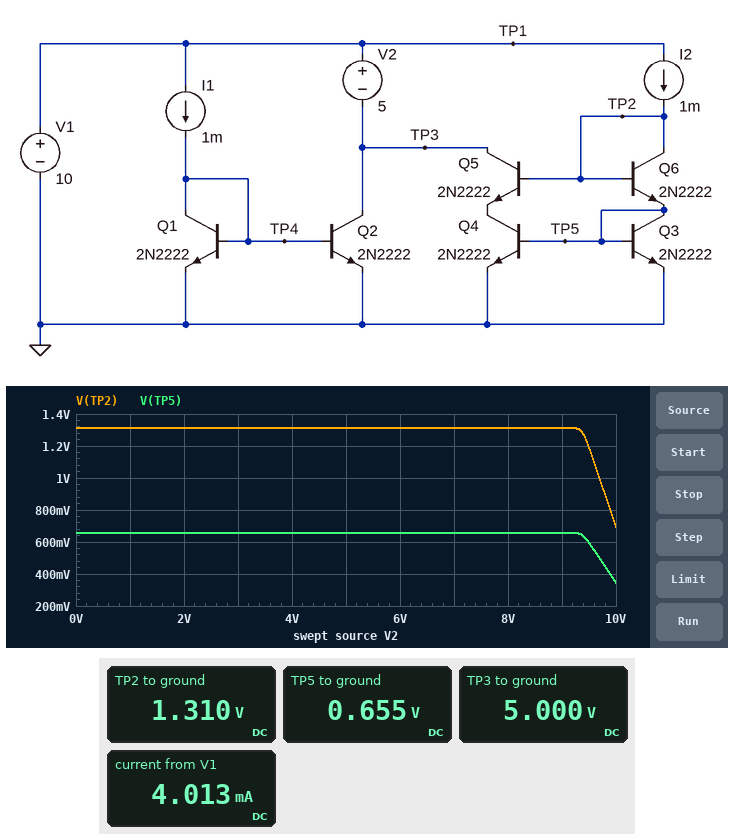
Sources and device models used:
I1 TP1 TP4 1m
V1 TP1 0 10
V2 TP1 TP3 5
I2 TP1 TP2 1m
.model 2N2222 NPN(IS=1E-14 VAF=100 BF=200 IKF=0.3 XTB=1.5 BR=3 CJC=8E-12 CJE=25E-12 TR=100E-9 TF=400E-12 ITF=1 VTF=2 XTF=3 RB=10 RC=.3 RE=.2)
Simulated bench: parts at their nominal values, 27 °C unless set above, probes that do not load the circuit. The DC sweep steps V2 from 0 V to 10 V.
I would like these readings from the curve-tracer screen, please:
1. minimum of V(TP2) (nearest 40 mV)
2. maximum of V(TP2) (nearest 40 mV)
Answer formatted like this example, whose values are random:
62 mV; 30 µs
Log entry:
680 mV; 1.32 V
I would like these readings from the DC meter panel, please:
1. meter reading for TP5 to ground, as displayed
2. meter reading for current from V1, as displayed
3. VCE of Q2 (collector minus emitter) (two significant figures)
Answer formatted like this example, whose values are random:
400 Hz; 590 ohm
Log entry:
0.655 V; 4.013 mA; 5.0 V
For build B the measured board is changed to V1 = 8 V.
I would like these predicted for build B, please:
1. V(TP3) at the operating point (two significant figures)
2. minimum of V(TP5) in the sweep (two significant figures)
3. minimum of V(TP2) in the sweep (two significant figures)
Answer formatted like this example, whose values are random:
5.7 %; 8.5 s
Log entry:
3.0 V; -1.6 V; -1.3 V
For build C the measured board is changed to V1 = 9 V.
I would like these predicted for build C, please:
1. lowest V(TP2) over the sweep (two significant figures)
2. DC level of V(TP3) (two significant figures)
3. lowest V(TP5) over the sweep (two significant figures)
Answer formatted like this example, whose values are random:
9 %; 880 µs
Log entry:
-310 mV; 4.0 V; -640 mV
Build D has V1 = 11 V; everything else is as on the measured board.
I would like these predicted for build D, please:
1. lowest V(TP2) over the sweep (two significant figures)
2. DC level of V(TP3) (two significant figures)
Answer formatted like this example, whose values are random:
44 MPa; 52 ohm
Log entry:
1.3 V; 6.0 V
